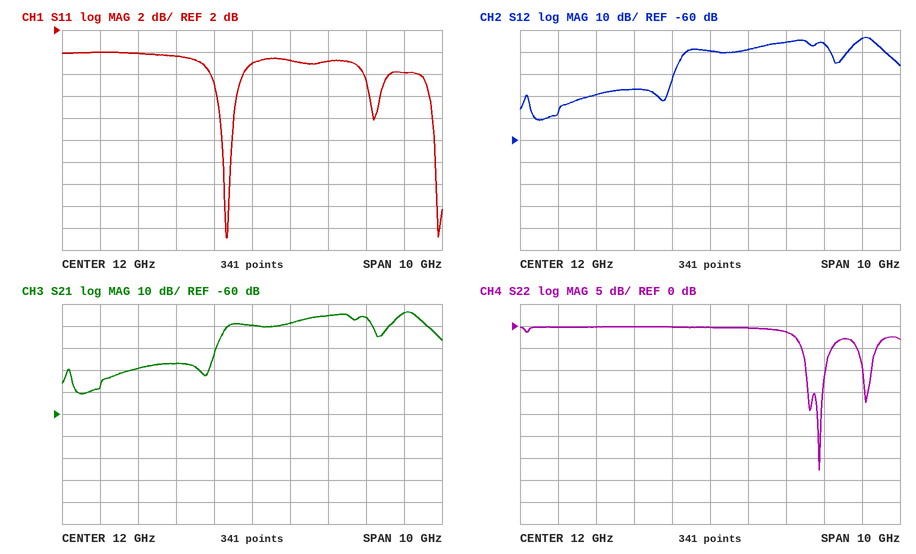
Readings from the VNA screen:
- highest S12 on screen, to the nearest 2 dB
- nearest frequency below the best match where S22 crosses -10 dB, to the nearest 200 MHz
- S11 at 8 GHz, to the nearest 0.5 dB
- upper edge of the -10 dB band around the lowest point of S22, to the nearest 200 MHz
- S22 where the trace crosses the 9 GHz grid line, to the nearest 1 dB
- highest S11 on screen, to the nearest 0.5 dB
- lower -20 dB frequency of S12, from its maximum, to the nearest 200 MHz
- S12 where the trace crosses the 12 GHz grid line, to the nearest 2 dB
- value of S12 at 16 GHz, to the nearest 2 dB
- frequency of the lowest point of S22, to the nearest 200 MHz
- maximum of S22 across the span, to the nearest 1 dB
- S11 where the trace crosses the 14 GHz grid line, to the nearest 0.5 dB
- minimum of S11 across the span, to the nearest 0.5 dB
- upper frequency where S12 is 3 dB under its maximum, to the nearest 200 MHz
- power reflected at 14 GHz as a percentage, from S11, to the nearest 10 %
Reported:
-14 dB
14.6 GHz
0.0 dB
15.0 GHz
0 dB
0.0 dB
11.0 GHz
-20 dB
-14 dB
14.8 GHz
0 dB
-1.0 dB
-17.0 dB
16.4 GHz
80 %
